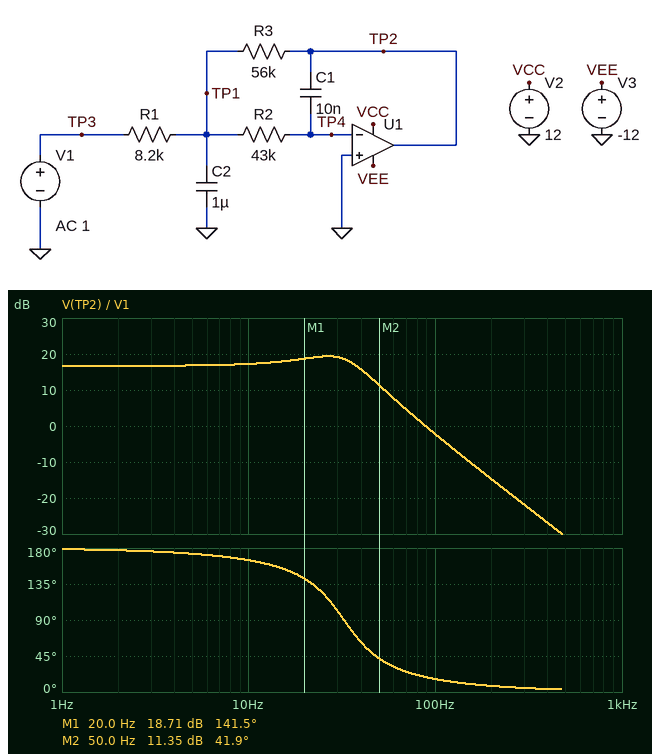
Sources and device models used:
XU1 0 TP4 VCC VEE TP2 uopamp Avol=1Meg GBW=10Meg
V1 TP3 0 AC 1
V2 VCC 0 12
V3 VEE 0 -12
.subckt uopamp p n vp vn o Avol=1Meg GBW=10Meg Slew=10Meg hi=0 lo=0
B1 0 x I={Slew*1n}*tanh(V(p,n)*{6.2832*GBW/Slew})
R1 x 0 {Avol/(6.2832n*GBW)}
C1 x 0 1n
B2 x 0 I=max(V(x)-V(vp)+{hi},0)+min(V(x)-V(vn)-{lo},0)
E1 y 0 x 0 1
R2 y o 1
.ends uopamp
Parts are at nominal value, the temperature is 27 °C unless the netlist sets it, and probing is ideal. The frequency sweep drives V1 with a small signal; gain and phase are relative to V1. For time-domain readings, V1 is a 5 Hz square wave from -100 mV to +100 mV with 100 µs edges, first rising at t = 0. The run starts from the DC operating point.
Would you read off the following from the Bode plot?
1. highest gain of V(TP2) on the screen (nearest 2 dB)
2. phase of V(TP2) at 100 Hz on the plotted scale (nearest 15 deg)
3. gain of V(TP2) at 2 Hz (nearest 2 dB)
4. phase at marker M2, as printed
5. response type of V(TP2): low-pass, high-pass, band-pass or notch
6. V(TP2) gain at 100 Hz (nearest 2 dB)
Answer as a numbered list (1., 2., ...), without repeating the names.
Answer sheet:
1. 20 dB
2. 15 deg
3. 16 dB
4. 41.9 deg
5. low-pass
6. -2 dB
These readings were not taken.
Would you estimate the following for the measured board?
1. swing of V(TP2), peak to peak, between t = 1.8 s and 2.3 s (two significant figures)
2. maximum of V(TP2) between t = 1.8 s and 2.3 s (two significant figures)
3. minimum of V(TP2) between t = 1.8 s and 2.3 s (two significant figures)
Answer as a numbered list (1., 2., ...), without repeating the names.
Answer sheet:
1. 2.1 V
2. 1.0 V
3. -1.0 V
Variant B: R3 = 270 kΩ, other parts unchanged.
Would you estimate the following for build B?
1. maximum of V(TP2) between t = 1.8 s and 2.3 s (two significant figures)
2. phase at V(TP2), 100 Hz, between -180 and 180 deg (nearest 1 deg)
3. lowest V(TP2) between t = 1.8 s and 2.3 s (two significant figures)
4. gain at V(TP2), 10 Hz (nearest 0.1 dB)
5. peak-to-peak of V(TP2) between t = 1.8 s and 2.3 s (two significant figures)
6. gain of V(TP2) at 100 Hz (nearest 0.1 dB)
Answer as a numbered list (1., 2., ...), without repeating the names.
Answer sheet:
1. 3.4 V
2. 14 deg
3. -3.4 V
4. 28.7 dB
5. 6.8 V
6. -2.9 dB
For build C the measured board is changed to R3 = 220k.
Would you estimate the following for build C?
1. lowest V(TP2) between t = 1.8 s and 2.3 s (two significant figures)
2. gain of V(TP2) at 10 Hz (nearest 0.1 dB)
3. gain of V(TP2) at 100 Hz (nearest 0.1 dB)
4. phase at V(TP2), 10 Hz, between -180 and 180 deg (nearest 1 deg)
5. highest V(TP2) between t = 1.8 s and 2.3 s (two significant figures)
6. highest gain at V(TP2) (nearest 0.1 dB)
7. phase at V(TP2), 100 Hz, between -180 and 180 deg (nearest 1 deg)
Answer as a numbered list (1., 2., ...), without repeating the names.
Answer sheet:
1. -2.9 V
2. 27.8 dB
3. -2.9 dB
4. 125 deg
5. 2.9 V
6. 28.6 dB
7. 14 deg
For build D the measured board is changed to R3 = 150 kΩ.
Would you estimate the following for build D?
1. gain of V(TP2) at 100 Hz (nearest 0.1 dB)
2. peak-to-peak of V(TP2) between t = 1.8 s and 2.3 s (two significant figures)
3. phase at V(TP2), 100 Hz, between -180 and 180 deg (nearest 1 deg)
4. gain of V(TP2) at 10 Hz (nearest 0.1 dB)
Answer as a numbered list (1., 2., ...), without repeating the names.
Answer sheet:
1. -2.8 dB
2. 4.3 V
3. 14 deg
4. 25.5 dB
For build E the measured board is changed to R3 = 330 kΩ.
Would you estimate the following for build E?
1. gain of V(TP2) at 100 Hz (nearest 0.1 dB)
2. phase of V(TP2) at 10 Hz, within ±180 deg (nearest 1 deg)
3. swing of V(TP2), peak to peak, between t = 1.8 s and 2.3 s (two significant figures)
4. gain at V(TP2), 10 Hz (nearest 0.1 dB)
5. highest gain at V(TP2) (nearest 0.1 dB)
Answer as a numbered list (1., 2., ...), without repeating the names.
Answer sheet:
1. -3.0 dB
2. 108 deg
3. 8.1 V
4. 29.2 dB
5. 32.1 dB
